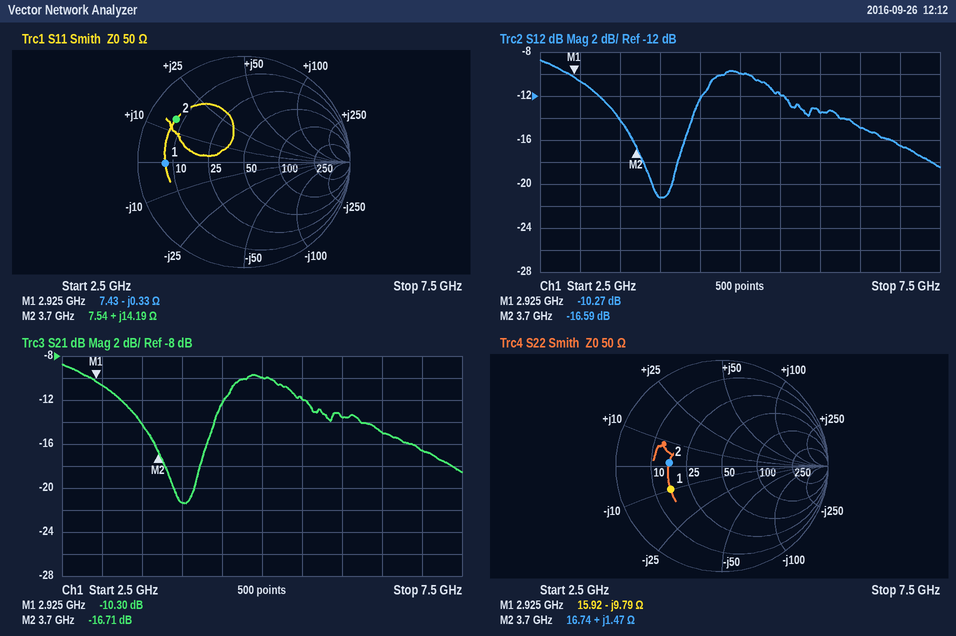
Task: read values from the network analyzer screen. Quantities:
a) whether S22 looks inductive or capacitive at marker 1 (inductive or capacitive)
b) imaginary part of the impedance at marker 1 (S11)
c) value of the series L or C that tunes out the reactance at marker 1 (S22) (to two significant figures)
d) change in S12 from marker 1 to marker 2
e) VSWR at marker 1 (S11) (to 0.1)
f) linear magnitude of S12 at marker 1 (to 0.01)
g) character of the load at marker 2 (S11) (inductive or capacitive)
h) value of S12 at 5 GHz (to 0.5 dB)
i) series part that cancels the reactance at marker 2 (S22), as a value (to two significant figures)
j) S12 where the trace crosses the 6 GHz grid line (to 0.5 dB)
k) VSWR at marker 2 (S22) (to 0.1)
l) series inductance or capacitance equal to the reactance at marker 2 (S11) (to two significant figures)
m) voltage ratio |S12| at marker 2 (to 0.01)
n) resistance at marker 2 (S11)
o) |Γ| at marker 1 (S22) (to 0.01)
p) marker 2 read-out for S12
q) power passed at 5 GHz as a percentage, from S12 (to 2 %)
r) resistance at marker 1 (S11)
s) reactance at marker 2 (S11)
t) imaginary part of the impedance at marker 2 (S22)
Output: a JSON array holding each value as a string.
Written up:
["capacitive", "-0.33 Ω", "530 pH", "-6.32 dB", "6.7", "0.31", "inductive", "-10.0 dB", "29 pF", "-13.5 dB", "3.0", "610 pH", "0.15", "7.54 Ω", "0.53", "-16.59 dB", "10 %", "7.43 Ω", "+14.19 Ω", "+1.47 Ω"]
